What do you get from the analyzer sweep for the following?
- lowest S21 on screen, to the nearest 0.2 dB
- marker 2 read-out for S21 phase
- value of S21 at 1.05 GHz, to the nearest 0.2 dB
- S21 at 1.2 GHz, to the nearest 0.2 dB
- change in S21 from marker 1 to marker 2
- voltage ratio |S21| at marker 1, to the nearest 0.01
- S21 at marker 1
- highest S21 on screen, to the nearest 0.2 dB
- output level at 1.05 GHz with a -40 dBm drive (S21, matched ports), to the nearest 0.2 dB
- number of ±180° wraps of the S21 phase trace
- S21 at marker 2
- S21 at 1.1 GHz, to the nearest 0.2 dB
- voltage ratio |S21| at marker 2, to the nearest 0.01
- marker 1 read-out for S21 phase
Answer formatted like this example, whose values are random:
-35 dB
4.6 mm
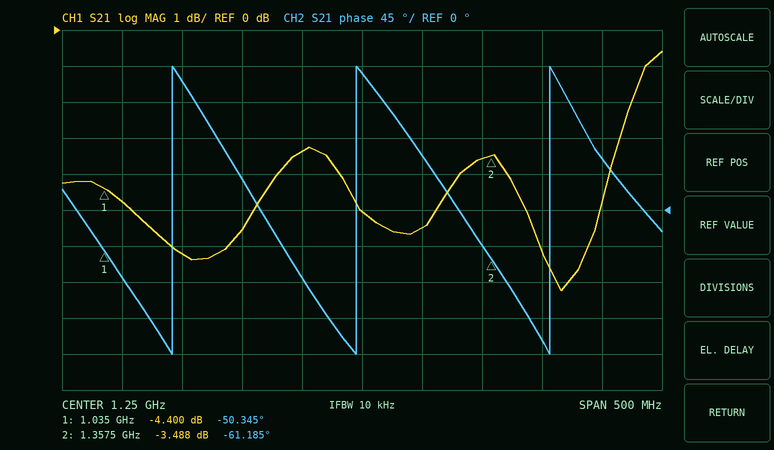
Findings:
-7.2 dB
-61.185°
-4.8 dB
-3.4 dB
0.912 dB
0.60
-4.400 dB
-0.6 dB
-44.8 dBm
3
-3.488 dB
-6.2 dB
0.67
-50.345°
